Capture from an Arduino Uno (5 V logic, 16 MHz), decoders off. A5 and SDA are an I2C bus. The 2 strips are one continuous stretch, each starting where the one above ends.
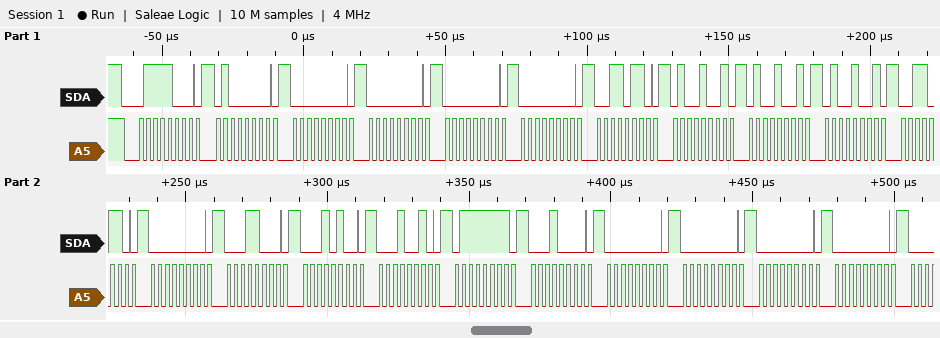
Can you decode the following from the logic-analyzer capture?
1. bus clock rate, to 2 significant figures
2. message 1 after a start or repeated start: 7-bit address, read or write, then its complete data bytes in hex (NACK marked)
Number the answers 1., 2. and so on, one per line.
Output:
1. 400 kHz
2. 0x3C write: 40 00 00 00 00 36 49 49 49 36 00 18 14 12 7F 10 00 00 00 00
